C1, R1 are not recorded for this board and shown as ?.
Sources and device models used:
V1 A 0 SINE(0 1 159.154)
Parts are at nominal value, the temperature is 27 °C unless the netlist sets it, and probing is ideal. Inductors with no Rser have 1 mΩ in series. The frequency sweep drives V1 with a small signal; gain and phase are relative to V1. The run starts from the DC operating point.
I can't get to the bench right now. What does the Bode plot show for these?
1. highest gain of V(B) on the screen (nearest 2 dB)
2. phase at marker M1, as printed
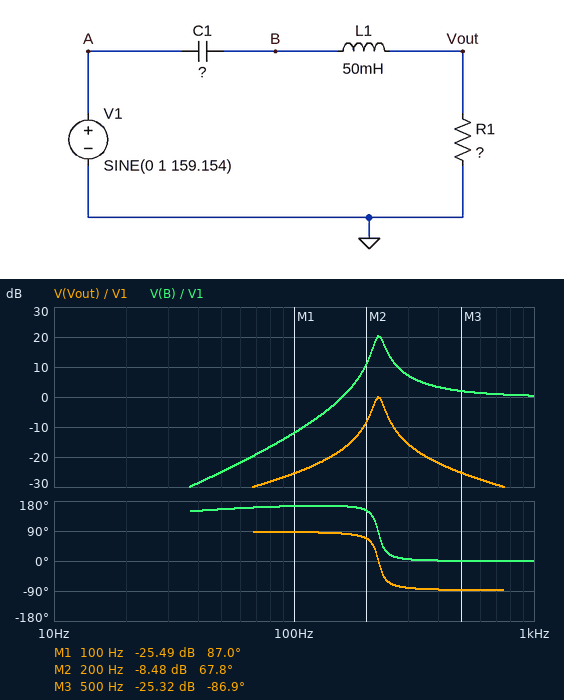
20 dB
87.0 deg
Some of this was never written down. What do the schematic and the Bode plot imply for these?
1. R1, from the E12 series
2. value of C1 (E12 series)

6.8 Ω
10 µF
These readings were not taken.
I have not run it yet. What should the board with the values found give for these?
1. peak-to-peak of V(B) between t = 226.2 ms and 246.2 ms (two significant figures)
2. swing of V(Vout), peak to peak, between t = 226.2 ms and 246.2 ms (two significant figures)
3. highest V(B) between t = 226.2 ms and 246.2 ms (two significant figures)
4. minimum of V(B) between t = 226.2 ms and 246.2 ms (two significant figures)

2.0 V
270 mV
1.0 V
-1.0 V
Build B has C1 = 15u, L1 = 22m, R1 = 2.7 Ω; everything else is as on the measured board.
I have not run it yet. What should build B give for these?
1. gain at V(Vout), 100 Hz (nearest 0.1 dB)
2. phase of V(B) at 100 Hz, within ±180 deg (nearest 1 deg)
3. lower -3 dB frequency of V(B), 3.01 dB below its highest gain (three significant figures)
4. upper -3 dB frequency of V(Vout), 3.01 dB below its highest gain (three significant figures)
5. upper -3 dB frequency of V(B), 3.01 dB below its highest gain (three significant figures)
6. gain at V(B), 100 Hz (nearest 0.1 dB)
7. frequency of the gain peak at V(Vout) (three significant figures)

-30.7 dB
167 deg
268 Hz
287 Hz
288 Hz
-16.3 dB
277 Hz
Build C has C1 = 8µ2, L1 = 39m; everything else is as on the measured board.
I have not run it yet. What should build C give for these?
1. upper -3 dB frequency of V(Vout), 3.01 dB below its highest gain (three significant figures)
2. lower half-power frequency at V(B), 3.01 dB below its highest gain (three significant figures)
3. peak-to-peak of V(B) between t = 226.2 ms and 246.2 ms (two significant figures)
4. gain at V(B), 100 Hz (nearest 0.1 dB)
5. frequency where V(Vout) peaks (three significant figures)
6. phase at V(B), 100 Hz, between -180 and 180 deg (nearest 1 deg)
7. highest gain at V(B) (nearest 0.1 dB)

296 Hz
269 Hz
950 mV
-16.5 dB
281 Hz
162 deg
20.2 dB
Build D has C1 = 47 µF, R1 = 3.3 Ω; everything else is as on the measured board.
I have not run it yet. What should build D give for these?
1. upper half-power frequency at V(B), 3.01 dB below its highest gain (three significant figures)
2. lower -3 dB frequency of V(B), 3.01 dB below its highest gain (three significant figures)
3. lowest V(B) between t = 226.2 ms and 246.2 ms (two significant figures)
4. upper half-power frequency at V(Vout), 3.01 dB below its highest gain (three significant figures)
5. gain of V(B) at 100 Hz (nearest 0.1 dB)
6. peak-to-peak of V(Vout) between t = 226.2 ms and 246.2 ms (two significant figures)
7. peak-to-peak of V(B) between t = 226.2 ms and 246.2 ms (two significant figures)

110 Hz
99.2 Hz
-1.7 V
109 Hz
17.7 dB
230 mV
3.5 V
